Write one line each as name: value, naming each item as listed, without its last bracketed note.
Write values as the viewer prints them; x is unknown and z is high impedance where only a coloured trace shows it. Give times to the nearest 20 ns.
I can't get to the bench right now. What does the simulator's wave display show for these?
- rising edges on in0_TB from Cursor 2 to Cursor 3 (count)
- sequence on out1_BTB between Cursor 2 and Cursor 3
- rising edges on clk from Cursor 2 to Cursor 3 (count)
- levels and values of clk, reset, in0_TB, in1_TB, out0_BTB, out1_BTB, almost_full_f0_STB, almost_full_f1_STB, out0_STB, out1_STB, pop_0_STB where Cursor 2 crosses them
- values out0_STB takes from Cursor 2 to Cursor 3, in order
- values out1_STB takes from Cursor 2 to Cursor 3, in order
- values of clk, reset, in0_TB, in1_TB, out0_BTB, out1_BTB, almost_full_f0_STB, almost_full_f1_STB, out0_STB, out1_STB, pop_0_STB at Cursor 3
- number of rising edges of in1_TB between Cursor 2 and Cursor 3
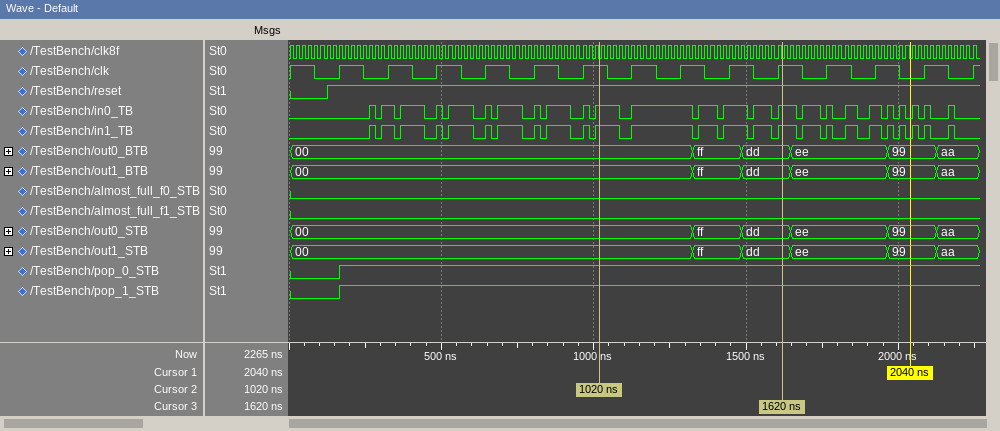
rising edges on in0_TB from Cursor 2 to Cursor 3: 5
sequence on out1_BTB between Cursor 2 and Cursor 3: 00, ff, dd
rising edges on clk from Cursor 2 to Cursor 3: 4
levels and values of clk, reset, in0_TB, in1_TB, out0_BTB, out1_BTB, almost_full_f0_STB, almost_full_f1_STB, out0_STB, out1_STB, pop_0_STB where Cursor 2 crosses them: clk=1, reset=1, in0_TB=1, in1_TB=1, out0_BTB=00, out1_BTB=00, almost_full_f0_STB=0, almost_full_f1_STB=0, out0_STB=00, out1_STB=00, pop_0_STB=1
values out0_STB takes from Cursor 2 to Cursor 3, in order: 00, ff, dd
values out1_STB takes from Cursor 2 to Cursor 3, in order: 00, ff, dd
values of clk, reset, in0_TB, in1_TB, out0_BTB, out1_BTB, almost_full_f0_STB, almost_full_f1_STB, out0_STB, out1_STB, pop_0_STB at Cursor 3: clk=1, reset=1, in0_TB=1, in1_TB=1, out0_BTB=dd, out1_BTB=dd, almost_full_f0_STB=0, almost_full_f1_STB=0, out0_STB=dd, out1_STB=dd, pop_0_STB=1
number of rising edges of in1_TB between Cursor 2 and Cursor 3: 5
